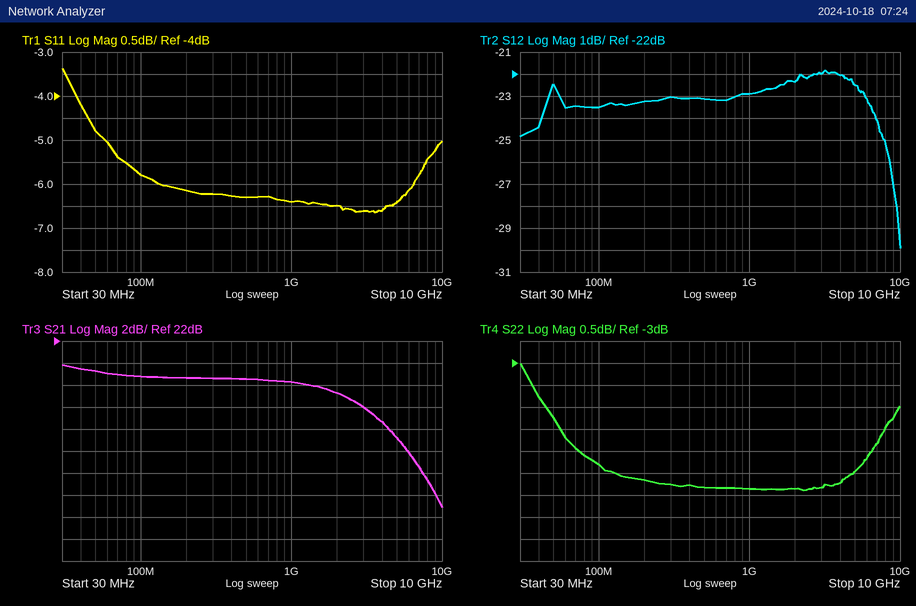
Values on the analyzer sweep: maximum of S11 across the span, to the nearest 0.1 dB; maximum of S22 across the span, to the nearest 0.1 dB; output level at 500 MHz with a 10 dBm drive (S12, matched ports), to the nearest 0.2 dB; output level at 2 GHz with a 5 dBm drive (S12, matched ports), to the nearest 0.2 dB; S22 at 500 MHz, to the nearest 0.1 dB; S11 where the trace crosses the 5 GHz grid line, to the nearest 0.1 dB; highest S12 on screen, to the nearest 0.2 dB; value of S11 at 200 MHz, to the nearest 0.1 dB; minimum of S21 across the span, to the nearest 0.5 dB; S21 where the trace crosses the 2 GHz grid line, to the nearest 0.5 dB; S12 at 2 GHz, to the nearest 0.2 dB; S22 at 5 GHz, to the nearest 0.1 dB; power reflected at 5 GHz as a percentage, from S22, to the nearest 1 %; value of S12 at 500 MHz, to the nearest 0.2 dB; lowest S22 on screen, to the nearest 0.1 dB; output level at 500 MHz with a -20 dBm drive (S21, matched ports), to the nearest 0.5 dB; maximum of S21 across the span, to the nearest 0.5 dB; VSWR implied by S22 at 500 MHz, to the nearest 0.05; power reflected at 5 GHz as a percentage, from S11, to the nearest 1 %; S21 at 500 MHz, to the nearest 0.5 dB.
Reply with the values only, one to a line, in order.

-3.4 dB
-3.0 dB
-13.2 dBm
-17.4 dBm
-5.8 dB
-6.4 dB
-21.8 dB
-6.1 dB
7.0 dB
17.5 dB
-22.4 dB
-5.5 dB
28 %
-23.2 dB
-5.9 dB
-1.5 dBm
20.0 dB
3.10
23 %
18.5 dB
